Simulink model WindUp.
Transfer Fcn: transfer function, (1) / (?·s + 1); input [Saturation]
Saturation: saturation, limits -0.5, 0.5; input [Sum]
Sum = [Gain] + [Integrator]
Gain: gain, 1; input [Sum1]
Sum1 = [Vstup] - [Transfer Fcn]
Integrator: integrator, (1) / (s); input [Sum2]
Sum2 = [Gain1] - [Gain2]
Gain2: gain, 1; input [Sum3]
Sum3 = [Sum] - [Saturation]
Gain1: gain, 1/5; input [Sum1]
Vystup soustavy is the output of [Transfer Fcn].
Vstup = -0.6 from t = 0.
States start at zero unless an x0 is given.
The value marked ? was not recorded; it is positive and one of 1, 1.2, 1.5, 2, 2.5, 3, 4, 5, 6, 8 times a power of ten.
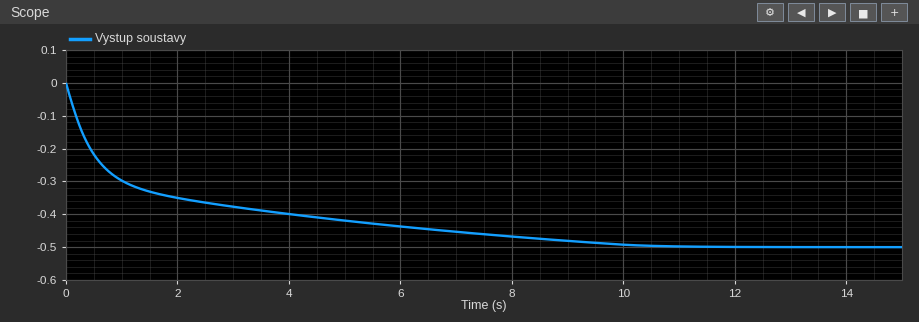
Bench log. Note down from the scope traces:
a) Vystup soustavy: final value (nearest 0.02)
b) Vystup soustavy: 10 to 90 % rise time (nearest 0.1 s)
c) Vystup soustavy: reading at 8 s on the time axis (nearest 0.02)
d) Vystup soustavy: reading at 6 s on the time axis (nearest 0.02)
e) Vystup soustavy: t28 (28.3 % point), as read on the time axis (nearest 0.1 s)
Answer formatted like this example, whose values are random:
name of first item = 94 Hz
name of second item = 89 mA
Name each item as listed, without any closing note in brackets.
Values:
Vystup soustavy: final value = -0.50
Vystup soustavy: 10 to 90 % rise time = 6.7 s
Vystup soustavy: reading at 8 s on the time axis = -0.46
Vystup soustavy: reading at 6 s on the time axis = -0.44
Vystup soustavy: t28 (28.3 % point), as read on the time axis = 0.3 s
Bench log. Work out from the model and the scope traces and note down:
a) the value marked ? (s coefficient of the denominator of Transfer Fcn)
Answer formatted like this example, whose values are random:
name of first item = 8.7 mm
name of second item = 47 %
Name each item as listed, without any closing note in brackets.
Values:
the value marked ? = 0.8
